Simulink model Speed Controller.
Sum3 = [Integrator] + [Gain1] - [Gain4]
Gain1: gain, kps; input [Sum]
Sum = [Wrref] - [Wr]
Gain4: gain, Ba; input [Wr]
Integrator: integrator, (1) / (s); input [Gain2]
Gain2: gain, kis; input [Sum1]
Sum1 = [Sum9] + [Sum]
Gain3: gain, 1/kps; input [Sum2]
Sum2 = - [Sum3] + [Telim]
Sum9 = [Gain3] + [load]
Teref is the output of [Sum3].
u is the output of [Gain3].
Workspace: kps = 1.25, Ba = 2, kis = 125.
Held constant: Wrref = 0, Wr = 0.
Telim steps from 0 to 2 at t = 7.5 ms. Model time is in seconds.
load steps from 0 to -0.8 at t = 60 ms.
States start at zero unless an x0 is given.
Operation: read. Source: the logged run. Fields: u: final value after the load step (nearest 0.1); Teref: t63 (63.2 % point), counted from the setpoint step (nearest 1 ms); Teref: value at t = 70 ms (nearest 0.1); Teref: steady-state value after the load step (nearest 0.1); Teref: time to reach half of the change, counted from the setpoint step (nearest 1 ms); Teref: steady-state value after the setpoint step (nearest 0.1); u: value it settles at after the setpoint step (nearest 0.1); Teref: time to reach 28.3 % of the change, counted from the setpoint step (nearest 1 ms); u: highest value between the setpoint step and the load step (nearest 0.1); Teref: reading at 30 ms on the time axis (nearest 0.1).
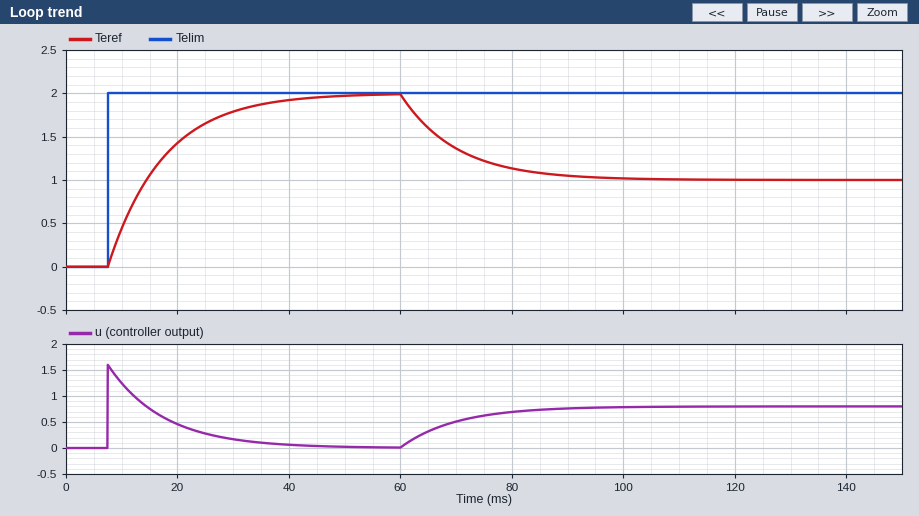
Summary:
0.8
10 ms
1.4
1.0
7 ms
2.0
0.0
3 ms
1.6
1.8
